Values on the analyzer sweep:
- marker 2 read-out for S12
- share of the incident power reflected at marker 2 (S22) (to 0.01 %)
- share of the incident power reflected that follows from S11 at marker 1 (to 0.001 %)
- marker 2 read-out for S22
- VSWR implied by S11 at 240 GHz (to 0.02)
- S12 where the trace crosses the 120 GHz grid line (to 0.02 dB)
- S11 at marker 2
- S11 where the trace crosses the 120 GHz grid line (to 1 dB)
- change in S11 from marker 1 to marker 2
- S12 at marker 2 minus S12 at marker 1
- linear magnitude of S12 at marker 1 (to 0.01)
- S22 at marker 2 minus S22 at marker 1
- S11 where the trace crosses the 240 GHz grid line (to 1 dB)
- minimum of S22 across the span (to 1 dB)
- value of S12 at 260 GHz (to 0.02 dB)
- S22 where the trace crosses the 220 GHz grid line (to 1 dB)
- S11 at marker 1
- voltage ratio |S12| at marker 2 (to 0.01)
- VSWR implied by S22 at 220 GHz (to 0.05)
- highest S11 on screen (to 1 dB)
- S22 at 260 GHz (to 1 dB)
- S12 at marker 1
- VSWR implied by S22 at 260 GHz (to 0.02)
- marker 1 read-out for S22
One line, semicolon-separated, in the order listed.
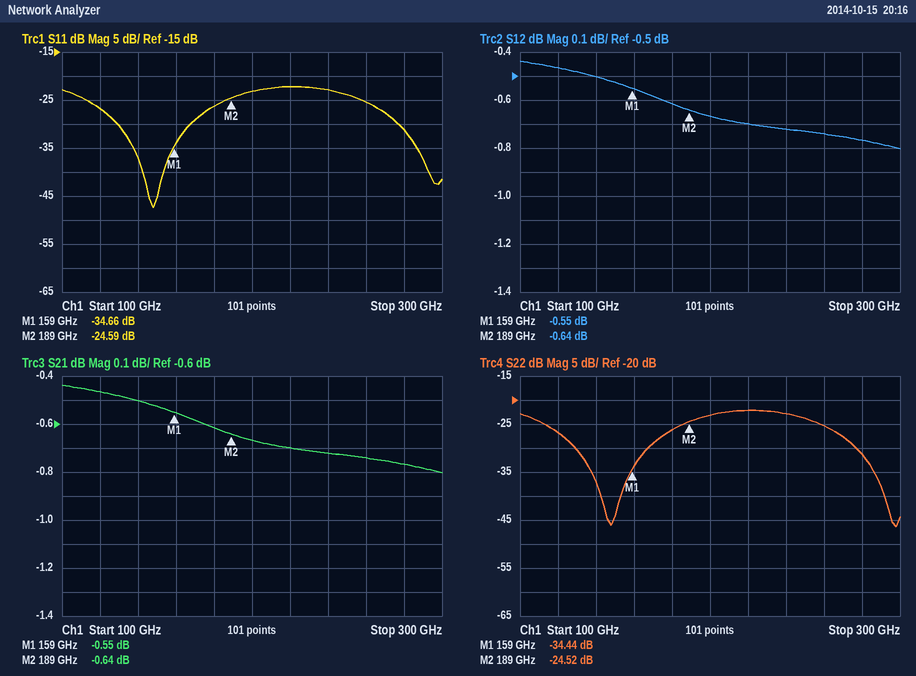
-0.64 dB; 0.35 %; 0.034 %; -24.52 dB; 1.16; -0.46 dB; -24.59 dB; -27 dB; 10.07 dB; -0.09 dB; 0.94; 9.92 dB; -23 dB; -46 dB; -0.74 dB; -22 dB; -34.66 dB; 0.93; 1.15; -22 dB; -25 dB; -0.55 dB; 1.12; -34.44 dB
